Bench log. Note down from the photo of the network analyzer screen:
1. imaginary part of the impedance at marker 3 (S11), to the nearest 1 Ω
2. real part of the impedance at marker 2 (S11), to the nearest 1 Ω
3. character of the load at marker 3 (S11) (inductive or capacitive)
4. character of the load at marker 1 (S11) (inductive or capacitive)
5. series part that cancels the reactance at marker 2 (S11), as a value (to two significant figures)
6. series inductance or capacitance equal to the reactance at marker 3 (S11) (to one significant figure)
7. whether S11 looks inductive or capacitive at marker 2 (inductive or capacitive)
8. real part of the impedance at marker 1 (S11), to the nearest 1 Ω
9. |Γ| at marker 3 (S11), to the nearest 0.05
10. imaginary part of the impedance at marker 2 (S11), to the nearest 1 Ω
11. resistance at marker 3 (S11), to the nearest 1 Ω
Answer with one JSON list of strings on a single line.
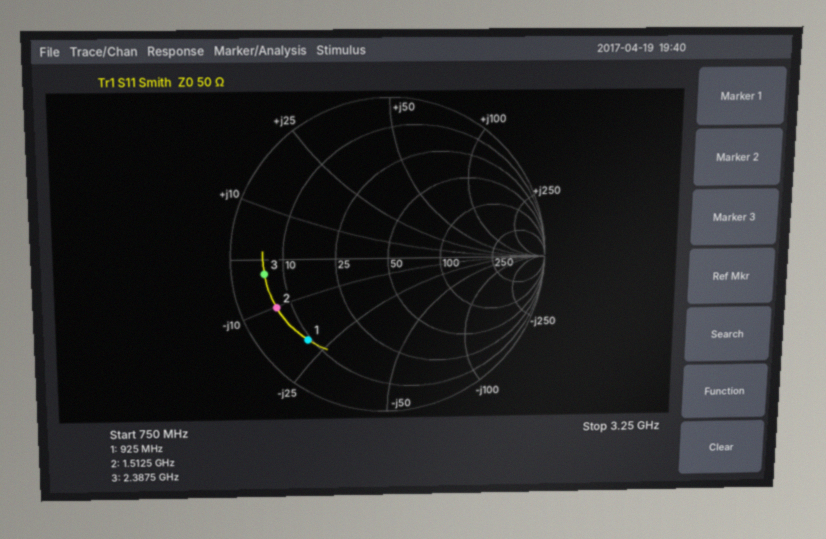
["-3 Ω", "7 Ω", "capacitive", "capacitive", "1.1 nH", "20 pF", "capacitive", "9 Ω", "0.80", "-10 Ω", "6 Ω"]
